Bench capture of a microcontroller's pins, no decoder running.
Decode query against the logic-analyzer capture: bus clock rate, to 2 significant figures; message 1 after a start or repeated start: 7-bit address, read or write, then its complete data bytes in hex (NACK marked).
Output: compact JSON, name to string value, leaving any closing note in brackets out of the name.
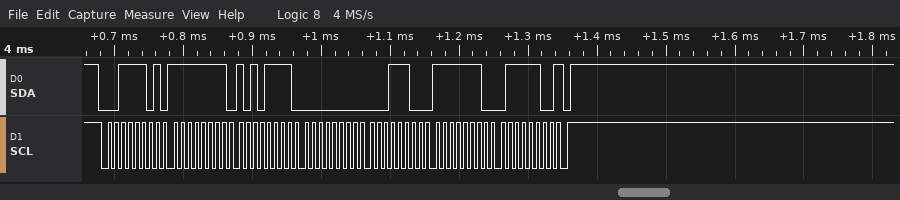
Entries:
{"bus clock rate, to 2 significant figures": "100 kHz", "message 1 after a start or repeated start: 7-bit address, read or write, then its complete data bytes in hex": "0x1E read: FF AF 00 1C FE 7C NACK"}
